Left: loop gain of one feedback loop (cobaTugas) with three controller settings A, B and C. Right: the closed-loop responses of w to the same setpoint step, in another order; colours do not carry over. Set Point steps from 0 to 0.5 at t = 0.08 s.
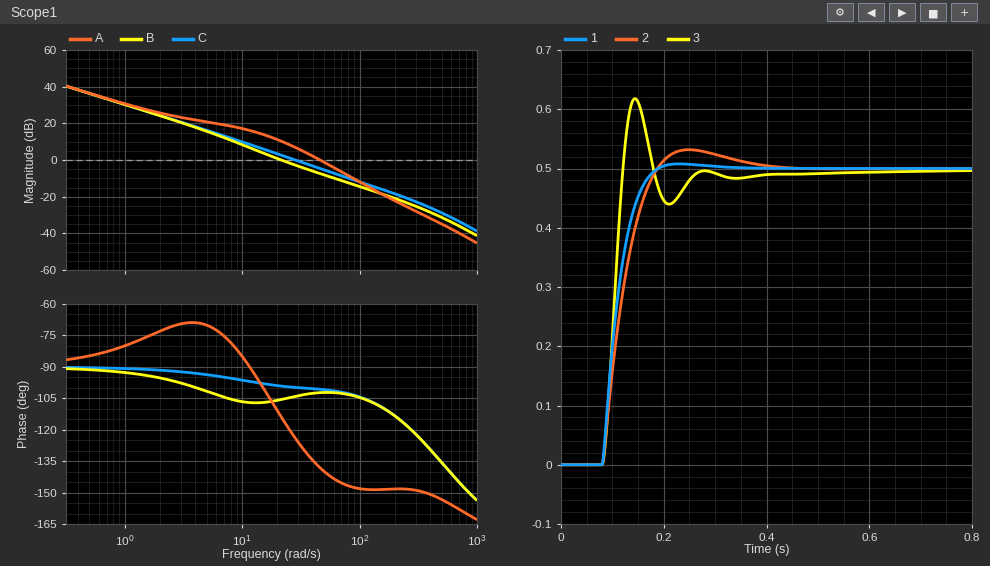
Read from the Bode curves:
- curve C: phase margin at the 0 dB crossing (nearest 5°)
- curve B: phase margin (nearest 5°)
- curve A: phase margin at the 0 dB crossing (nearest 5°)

80°
75°
40°
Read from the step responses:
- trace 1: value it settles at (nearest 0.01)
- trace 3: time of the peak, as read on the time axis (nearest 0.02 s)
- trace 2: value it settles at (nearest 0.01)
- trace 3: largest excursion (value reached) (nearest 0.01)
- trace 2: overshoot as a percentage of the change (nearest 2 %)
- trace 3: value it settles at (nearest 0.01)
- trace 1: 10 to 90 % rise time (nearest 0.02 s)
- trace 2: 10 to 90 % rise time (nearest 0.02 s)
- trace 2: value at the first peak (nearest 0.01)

0.50
0.14 s
0.50
0.62
6 %
0.50
0.06 s
0.08 s
0.53
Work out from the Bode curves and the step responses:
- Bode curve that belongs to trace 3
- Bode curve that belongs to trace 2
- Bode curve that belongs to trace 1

A
B
C
